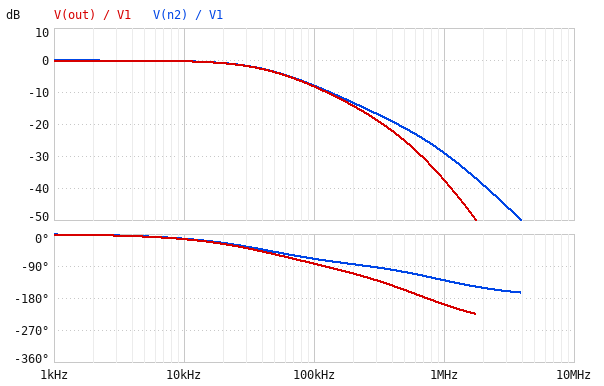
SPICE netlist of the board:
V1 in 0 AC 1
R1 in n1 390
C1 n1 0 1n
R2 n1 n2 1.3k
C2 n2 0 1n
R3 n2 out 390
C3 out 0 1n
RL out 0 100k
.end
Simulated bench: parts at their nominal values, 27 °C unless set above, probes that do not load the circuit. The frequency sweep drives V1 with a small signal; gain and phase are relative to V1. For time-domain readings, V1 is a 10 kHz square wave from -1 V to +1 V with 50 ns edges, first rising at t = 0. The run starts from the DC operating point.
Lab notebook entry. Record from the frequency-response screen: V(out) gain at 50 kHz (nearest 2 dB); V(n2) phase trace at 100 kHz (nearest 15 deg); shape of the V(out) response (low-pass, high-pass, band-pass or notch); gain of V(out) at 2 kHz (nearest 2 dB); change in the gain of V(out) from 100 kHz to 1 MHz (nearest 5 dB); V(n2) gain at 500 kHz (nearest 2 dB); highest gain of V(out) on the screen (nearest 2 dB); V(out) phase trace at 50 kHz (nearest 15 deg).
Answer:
-4 dB
-75 deg
low-pass
0 dB
-30 dB
-22 dB
0 dB
-60 deg
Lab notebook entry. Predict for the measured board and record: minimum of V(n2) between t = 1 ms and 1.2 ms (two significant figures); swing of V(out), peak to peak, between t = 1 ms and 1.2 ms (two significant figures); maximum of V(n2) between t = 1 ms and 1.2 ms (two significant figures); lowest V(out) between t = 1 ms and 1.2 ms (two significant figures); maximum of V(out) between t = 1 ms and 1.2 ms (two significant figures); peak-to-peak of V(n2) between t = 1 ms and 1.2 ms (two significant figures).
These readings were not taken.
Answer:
-980 mV
2.0 V
980 mV
-980 mV
980 mV
2.0 V
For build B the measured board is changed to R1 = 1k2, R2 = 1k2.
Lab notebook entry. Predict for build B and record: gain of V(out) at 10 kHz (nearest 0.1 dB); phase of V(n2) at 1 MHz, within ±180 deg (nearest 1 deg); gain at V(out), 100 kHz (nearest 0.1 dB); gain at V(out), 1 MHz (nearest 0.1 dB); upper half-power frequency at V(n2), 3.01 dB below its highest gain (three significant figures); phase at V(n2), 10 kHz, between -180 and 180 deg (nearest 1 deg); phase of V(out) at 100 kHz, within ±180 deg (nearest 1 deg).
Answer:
-0.7 dB
-143 deg
-11.9 dB
-45.8 dB
28.7 kHz
-20 deg
-100 deg
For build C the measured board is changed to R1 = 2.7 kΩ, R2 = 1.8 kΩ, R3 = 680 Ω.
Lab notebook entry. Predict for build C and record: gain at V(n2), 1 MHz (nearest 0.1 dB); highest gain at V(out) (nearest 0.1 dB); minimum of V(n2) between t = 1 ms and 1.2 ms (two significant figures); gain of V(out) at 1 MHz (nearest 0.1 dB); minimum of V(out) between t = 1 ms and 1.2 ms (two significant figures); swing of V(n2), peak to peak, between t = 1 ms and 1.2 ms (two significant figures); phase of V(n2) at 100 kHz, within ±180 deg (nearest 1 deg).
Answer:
-46.6 dB
-0.4 dB
-940 mV
-59.5 dB
-930 mV
1.9 V
-101 deg
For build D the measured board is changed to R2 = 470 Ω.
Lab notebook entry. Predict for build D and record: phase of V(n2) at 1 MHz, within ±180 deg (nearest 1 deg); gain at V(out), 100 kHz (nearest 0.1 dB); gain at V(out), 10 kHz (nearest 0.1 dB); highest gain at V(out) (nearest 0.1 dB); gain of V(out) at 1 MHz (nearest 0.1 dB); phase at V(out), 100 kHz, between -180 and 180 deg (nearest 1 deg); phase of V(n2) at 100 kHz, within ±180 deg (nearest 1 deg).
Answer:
-116 deg
-4.6 dB
-0.2 dB
-0.1 dB
-30.3 dB
-67 deg
-53 deg
